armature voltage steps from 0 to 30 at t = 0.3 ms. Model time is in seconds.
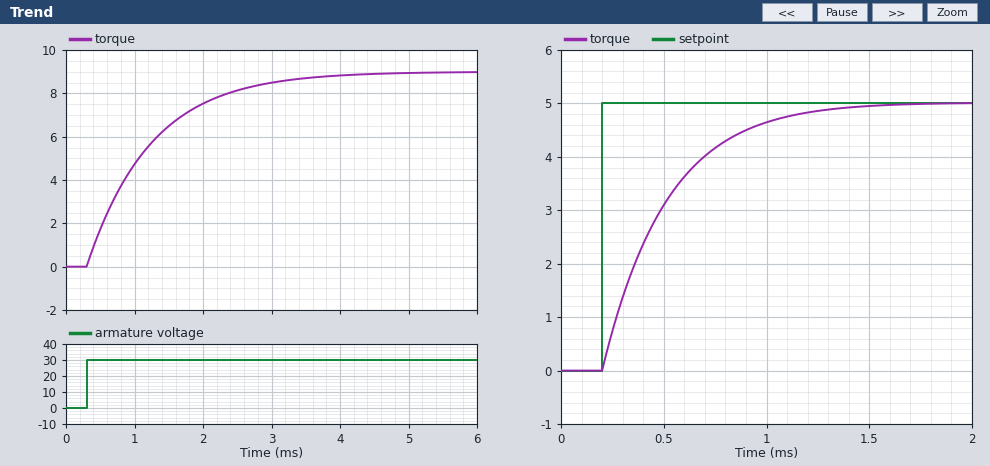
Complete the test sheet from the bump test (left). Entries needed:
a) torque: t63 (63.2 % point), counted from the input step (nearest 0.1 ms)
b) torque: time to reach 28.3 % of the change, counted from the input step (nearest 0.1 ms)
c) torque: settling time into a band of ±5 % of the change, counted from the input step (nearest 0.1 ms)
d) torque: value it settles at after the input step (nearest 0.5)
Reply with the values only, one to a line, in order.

0.9 ms
0.3 ms
2.8 ms
9.0
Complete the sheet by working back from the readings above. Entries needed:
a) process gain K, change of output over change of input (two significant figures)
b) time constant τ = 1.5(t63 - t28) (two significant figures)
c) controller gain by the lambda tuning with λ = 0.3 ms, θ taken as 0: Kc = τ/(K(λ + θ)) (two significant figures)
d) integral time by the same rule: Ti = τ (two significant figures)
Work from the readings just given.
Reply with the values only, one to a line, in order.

0.30
0.90 ms
10
0.90 ms
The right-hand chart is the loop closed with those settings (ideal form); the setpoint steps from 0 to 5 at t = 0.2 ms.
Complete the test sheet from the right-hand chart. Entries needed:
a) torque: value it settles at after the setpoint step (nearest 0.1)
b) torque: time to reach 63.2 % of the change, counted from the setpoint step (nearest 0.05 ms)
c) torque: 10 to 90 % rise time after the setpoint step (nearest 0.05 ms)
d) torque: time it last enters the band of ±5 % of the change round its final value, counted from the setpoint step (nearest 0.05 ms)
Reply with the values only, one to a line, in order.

5.0
0.30 ms
0.65 ms
0.90 ms
